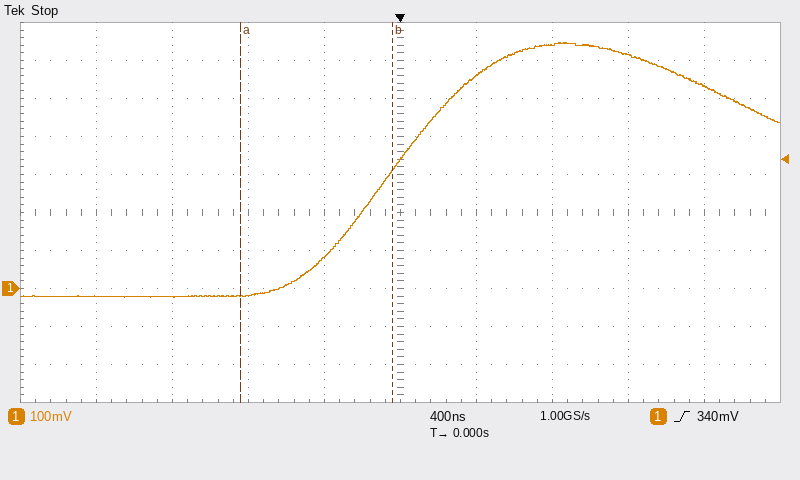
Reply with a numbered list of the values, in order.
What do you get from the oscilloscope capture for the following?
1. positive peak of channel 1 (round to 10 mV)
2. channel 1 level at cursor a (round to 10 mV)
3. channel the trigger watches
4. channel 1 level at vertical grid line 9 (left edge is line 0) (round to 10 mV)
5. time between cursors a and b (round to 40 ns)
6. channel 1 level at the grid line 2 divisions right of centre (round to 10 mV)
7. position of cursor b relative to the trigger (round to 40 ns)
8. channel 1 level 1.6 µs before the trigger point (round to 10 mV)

1. 650 mV
2. -20 mV
3. channel 1
4. 530 mV
5. 800 ns
6. 640 mV
7. -40 ns
8. -20 mV
